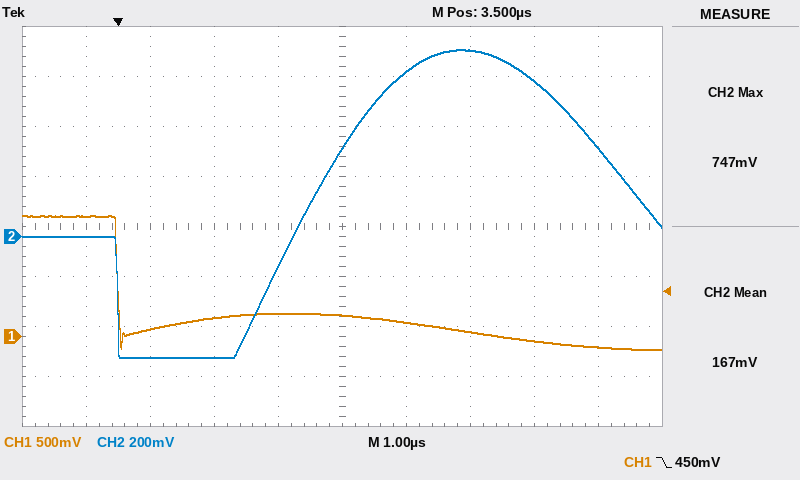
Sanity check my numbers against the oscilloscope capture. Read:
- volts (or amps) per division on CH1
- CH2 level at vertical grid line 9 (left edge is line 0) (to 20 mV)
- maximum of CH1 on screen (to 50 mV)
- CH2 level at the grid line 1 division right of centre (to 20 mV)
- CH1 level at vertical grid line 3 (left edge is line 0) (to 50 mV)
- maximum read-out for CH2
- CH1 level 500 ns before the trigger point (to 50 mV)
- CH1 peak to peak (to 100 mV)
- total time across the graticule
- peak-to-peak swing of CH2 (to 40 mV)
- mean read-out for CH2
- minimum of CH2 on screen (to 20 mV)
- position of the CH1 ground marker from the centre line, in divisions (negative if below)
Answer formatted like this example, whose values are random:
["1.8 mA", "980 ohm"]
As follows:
["500 mV", "360 mV", "1.20 V", "660 mV", "200 mV", "747 mV", "1.20 V", "1.30 V", "10 µs", "1.24 V", "167 mV", "-480 mV", "-2.2 div"]
